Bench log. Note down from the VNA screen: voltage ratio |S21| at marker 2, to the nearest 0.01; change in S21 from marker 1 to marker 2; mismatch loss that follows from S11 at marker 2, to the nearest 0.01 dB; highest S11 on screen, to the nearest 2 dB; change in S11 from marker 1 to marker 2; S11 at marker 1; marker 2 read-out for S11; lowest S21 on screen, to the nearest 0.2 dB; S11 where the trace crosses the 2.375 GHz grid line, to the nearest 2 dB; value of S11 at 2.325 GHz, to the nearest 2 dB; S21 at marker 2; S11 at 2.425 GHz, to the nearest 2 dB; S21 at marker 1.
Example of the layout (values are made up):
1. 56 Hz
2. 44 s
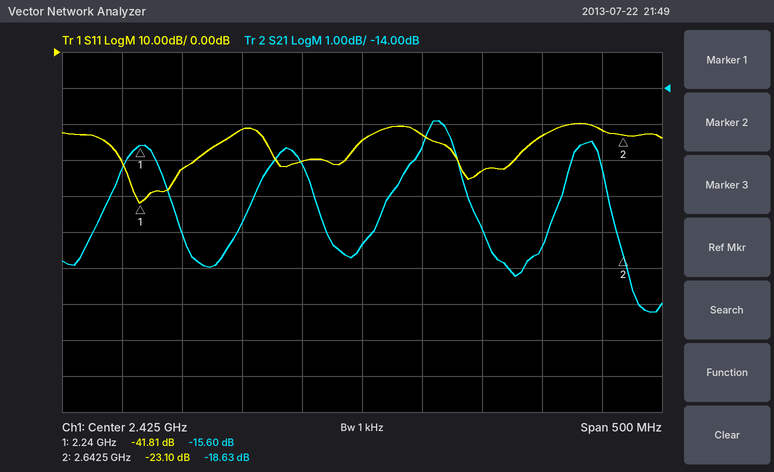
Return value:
1. 0.12
2. -3.03 dB
3. 0.02 dB
4. -20 dB
5. 18.71 dB
6. -41.81 dB
7. -23.10 dB
8. -20.2 dB
9. -30 dB
10. -22 dB
11. -18.63 dB
12. -24 dB
13. -15.60 dB
